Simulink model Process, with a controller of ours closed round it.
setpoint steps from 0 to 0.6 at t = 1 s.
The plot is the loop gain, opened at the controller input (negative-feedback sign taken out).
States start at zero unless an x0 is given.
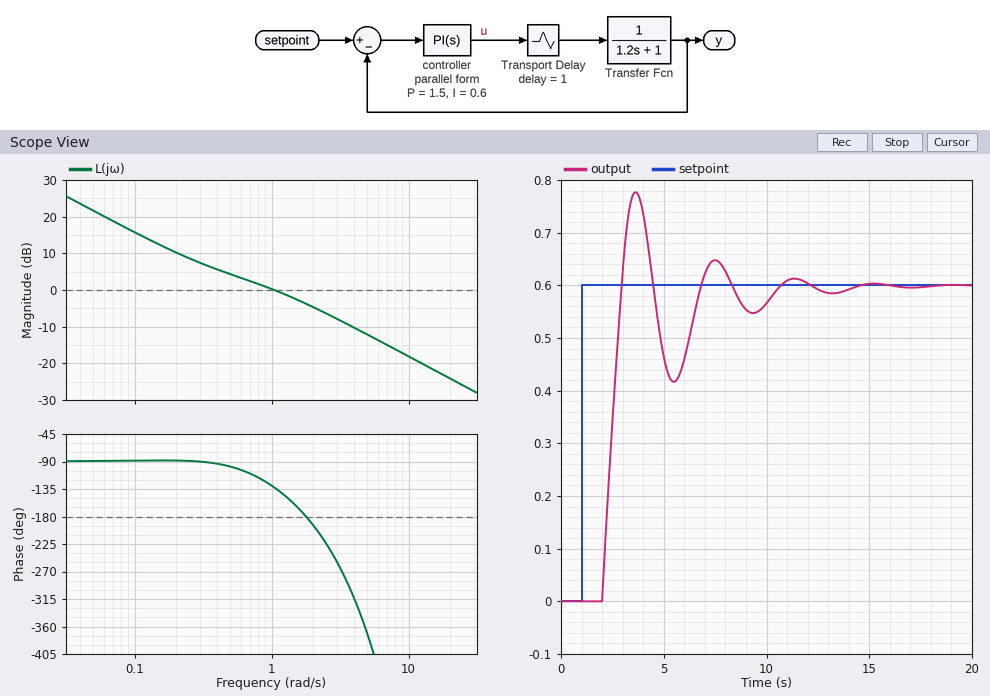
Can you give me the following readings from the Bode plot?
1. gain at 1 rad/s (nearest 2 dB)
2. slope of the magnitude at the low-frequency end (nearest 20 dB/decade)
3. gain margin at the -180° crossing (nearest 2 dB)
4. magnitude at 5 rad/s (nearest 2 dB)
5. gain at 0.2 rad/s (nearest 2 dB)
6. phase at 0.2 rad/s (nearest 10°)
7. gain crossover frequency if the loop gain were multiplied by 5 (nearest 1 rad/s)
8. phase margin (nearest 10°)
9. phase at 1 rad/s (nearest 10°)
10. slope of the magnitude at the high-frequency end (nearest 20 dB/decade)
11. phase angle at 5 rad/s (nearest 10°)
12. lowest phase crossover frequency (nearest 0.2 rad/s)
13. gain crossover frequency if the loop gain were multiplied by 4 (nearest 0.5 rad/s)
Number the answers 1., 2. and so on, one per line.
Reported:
1. 0 dB
2. -20 dB/decade
3. 4 dB
4. -12 dB
5. 10 dB
6. -90°
7. 6 rad/s
8. 50°
9. -130°
10. -20 dB/decade
11. -370°
12. 1.8 rad/s
13. 5.0 rad/s
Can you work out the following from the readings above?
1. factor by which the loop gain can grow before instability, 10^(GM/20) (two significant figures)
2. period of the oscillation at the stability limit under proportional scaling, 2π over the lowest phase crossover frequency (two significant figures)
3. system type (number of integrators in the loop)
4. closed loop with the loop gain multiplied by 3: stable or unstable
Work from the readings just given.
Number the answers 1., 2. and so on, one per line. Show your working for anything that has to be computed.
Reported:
1. 10^(4 / 20) = 1.6
2. 2π / 1.8 = 3.5 s
3. 1
4. unstable
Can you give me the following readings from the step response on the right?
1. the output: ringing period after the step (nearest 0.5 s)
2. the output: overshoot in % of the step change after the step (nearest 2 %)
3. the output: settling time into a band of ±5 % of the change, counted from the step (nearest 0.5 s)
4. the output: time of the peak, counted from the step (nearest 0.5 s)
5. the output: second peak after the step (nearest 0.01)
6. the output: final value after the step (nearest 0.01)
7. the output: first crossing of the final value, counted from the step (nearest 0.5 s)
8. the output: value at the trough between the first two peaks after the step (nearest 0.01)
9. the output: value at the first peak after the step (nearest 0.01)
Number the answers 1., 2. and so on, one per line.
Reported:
1. 4.0 s
2. 30 %
3. 9.0 s
4. 2.5 s
5. 0.65
6. 0.60
7. 2.0 s
8. 0.42
9. 0.78
